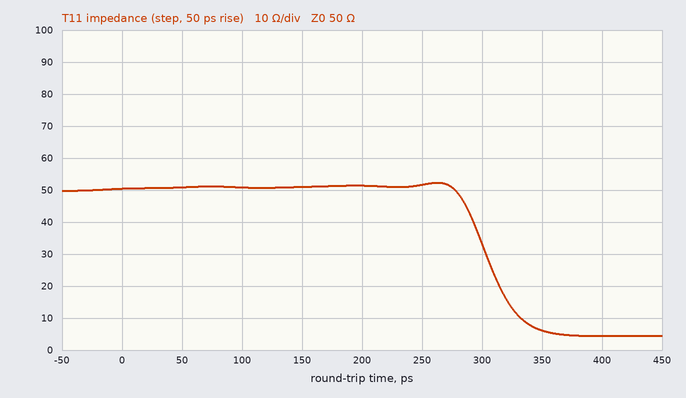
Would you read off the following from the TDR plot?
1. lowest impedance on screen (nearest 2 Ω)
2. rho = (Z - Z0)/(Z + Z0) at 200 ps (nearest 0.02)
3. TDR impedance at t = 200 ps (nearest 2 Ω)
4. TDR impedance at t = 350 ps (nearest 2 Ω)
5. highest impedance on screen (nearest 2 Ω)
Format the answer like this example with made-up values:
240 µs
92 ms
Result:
4 Ω
+0.02
52 Ω
6 Ω
52 Ω
